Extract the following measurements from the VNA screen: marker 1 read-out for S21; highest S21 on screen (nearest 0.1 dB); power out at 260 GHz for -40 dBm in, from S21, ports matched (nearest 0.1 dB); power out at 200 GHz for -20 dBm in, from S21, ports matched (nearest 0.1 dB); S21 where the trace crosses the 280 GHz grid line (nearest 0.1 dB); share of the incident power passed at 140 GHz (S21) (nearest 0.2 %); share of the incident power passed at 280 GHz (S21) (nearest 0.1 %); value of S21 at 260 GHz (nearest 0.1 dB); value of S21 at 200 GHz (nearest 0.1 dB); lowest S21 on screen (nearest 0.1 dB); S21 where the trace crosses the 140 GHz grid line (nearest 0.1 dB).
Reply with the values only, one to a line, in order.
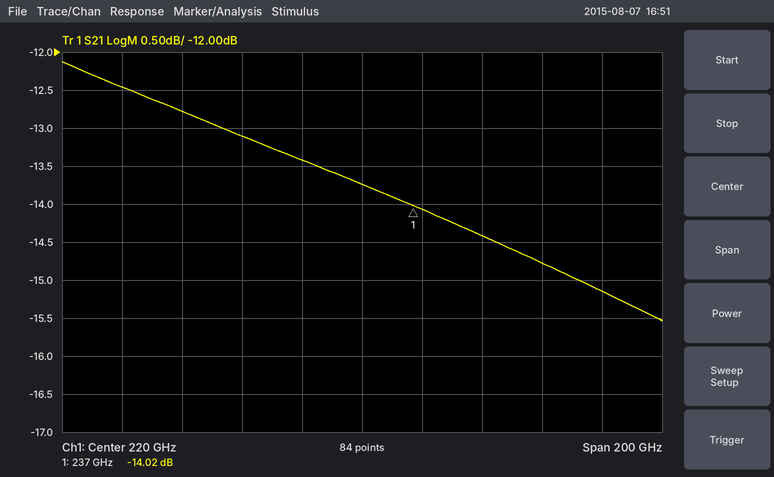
-14.02 dB
-12.1 dB
-54.4 dBm
-33.4 dBm
-14.8 dB
5.6 %
3.3 %
-14.4 dB
-13.4 dB
-15.5 dB
-12.5 dB
